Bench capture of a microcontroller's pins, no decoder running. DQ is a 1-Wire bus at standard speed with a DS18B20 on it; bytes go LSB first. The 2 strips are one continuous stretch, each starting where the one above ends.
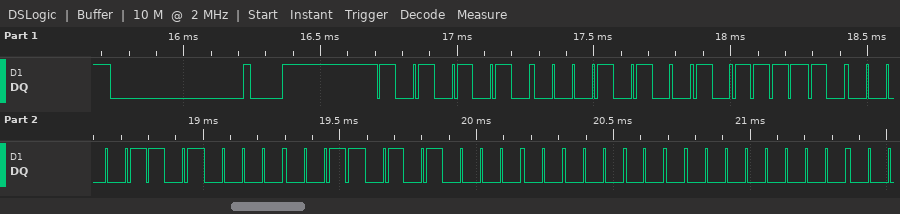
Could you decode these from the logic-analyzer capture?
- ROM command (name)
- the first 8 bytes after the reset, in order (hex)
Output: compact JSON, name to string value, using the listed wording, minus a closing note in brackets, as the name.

{"ROM command": "Match ROM", "the first 8 bytes after the reset, in order": "55 28 7D B0 C0 0A 00 00"}
